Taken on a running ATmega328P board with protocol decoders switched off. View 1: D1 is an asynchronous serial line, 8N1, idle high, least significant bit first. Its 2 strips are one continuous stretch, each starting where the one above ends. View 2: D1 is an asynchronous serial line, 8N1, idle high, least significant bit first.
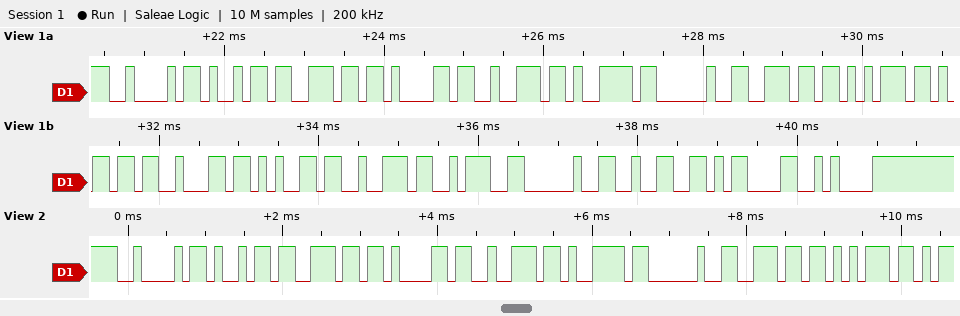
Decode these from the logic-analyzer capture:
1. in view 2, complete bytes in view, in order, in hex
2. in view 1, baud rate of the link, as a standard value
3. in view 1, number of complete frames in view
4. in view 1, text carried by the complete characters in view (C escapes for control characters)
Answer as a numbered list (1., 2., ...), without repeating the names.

1. 0x42 0x69 0x6E 0x61 0x72 0x79 0x20 0x6E 0x75
2. 9600 baud
3. 18
4. "Binary number: 2\r\n"
